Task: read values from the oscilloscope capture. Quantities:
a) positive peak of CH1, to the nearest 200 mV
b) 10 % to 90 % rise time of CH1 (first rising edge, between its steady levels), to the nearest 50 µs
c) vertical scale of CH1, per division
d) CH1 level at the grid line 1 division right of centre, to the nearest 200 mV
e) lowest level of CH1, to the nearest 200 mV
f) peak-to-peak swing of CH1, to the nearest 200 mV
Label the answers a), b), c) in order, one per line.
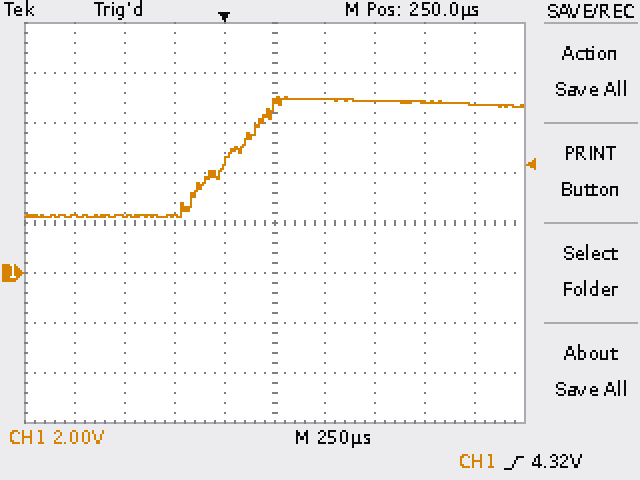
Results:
a) 7.0 V
b) 400 µs
c) 2 V
d) 7.0 V
e) 2.2 V
f) 4.8 V
